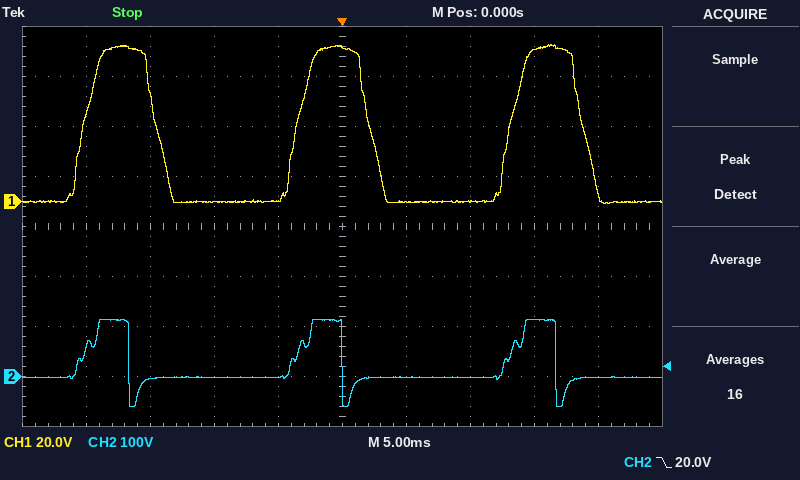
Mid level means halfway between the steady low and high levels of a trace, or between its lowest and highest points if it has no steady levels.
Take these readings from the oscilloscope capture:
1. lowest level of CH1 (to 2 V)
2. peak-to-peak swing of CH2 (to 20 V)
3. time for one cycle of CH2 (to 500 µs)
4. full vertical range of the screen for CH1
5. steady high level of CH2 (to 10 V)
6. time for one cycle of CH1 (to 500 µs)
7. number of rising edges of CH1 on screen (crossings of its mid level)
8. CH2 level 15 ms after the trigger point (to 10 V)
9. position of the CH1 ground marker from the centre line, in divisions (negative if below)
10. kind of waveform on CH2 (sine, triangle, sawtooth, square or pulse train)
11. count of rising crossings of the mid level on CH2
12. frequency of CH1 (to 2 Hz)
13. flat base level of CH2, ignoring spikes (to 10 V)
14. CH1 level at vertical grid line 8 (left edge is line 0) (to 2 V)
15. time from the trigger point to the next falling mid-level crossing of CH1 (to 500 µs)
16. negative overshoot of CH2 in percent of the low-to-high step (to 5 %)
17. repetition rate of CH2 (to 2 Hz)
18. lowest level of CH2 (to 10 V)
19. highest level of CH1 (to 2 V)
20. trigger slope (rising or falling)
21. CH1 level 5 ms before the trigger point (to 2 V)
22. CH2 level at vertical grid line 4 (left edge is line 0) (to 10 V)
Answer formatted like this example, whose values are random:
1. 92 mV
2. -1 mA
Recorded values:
1. 0 V
2. 180 V
3. 16.5 ms
4. 160 V
5. 110 V
6. 16.5 ms
7. 3
8. 110 V
9. +0.5 div
10. pulse train
11. 3
12. 60 Hz
13. 0 V
14. 60 V
15. 2.0 ms
16. 50 %
17. 60 Hz
18. -60 V
19. 62 V
20. falling
21. 0 V
22. 0 V
